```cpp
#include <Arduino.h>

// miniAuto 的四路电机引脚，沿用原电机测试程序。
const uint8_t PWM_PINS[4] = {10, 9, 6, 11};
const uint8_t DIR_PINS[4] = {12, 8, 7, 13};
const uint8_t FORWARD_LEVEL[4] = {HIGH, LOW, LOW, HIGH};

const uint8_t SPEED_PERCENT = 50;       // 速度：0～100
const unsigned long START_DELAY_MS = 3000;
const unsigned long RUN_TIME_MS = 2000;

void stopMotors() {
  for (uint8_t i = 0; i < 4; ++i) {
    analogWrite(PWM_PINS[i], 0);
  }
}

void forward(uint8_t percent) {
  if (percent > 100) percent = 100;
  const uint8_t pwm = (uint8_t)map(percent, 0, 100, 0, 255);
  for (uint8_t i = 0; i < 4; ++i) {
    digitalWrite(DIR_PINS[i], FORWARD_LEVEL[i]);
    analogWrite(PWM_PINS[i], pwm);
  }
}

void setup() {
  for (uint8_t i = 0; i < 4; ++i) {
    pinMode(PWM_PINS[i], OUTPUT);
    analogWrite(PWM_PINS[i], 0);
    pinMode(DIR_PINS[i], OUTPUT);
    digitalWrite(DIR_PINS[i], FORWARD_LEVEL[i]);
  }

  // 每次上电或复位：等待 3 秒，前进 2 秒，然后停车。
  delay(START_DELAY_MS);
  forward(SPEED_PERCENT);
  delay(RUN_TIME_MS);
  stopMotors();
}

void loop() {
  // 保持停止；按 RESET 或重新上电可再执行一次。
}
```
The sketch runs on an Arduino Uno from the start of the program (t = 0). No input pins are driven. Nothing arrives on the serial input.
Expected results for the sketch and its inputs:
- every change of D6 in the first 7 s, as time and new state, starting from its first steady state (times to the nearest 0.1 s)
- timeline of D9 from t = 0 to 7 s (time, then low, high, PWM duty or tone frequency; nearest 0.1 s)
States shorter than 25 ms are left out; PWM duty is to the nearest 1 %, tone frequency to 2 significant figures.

0 s low; 3 s PWM 50 %; 5 s low
0 s low; 3 s PWM 50 %; 5 s low
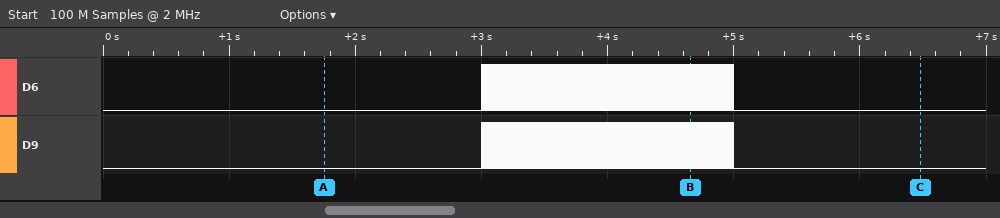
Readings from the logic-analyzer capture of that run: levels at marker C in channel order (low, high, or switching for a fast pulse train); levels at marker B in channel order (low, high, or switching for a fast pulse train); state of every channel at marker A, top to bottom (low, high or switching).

D6 low, D9 low
D6 switching, D9 switching
D6 low, D9 low
